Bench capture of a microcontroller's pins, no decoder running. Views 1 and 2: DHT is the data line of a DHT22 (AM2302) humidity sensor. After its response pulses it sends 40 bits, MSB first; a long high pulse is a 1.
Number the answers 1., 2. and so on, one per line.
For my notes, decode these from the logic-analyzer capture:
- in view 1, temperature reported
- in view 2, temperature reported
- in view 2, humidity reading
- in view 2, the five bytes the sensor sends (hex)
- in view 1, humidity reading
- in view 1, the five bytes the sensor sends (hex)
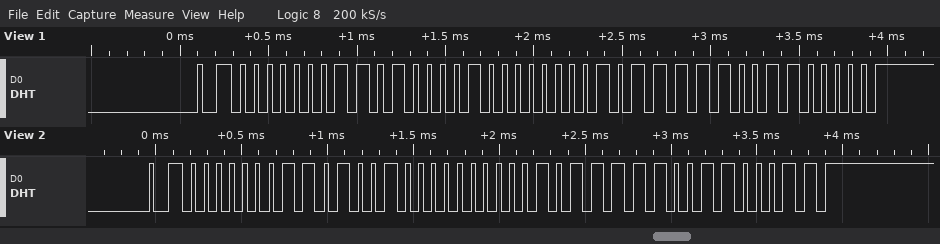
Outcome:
1. 19.0 °C
2. 19.0 °C
3. 42.0 %
4. 01 A4 00 BE 63
5. 41.7 %
6. 01 A1 00 BE 60
